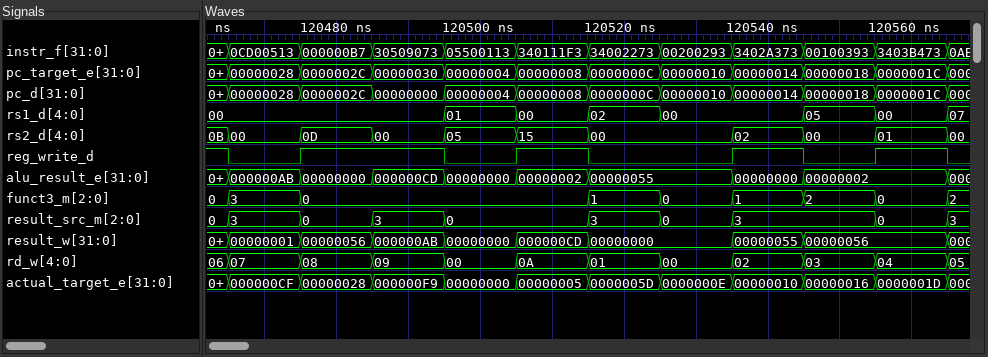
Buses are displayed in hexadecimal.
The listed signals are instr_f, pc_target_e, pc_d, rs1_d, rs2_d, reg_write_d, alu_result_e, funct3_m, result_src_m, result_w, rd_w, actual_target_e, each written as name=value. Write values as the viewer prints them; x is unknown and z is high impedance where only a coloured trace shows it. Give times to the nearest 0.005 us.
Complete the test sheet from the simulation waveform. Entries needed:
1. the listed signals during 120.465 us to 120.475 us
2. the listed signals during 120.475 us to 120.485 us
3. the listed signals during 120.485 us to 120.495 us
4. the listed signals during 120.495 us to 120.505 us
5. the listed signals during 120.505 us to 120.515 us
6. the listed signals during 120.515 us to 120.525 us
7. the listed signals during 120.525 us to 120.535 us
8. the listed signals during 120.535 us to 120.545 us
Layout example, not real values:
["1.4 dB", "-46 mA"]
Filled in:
["instr_f=0CD00513, pc_target_e=00000028, pc_d=00000028, rs1_d=00, rs2_d=00, reg_write_d=0, alu_result_e=000000AB, funct3_m=3, result_src_m=3, result_w=00000001, rd_w=07, actual_target_e=000000CF", "instr_f=000000B7, pc_target_e=0000002C, pc_d=0000002C, rs1_d=00, rs2_d=0D, reg_write_d=1, alu_result_e=00000000, funct3_m=0, result_src_m=0, result_w=00000056, rd_w=08, actual_target_e=00000028", "instr_f=30509073, pc_target_e=00000030, pc_d=00000000, rs1_d=00, rs2_d=00, reg_write_d=1, alu_result_e=000000CD, funct3_m=0, result_src_m=3, result_w=000000AB, rd_w=09, actual_target_e=000000F9", "instr_f=05500113, pc_target_e=00000004, pc_d=00000004, rs1_d=01, rs2_d=05, reg_write_d=0, alu_result_e=00000000, funct3_m=0, result_src_m=0, result_w=00000000, rd_w=00, actual_target_e=00000000", "instr_f=340111F3, pc_target_e=00000008, pc_d=00000008, rs1_d=00, rs2_d=15, reg_write_d=1, alu_result_e=00000002, funct3_m=0, result_src_m=0, result_w=000000CD, rd_w=0A, actual_target_e=00000005", "instr_f=34002273, pc_target_e=0000000C, pc_d=0000000C, rs1_d=02, rs2_d=00, reg_write_d=0, alu_result_e=00000055, funct3_m=1, result_src_m=3, result_w=00000000, rd_w=01, actual_target_e=0000005D", "instr_f=00200293, pc_target_e=00000010, pc_d=00000010, rs1_d=00, rs2_d=00, reg_write_d=0, alu_result_e=00000055, funct3_m=0, result_src_m=0, result_w=00000000, rd_w=00, actual_target_e=0000000E", "instr_f=3402A373, pc_target_e=00000014, pc_d=00000014, rs1_d=00, rs2_d=02, reg_write_d=1, alu_result_e=00000000, funct3_m=1, result_src_m=3, result_w=00000055, rd_w=02, actual_target_e=00000010"]
